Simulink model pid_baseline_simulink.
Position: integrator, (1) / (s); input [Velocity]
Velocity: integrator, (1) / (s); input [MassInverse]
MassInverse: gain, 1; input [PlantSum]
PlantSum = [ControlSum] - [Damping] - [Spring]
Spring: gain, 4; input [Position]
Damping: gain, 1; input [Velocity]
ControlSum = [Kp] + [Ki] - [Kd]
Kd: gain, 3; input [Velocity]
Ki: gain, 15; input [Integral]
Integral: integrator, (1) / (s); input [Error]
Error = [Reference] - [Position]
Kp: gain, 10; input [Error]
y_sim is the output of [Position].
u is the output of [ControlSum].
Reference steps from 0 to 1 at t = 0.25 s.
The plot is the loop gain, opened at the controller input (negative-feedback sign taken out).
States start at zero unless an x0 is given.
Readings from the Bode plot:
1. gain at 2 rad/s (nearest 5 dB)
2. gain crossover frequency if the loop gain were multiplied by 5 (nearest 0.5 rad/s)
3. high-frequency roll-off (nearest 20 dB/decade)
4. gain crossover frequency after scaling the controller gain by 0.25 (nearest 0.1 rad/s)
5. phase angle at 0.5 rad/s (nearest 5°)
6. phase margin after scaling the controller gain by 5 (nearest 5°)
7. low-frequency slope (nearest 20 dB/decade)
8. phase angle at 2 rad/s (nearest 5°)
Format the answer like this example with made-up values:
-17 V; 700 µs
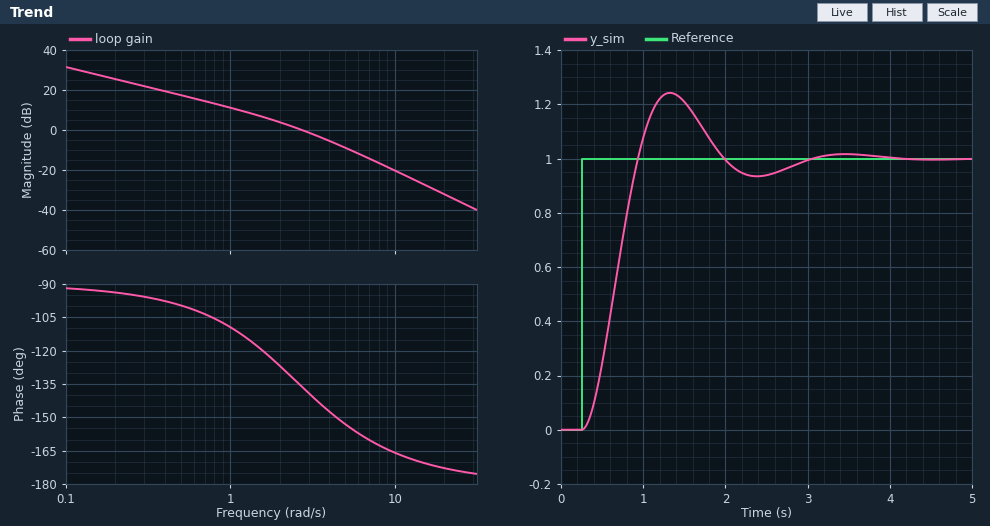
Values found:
5 dB; 7.0 rad/s; -40 dB/decade; 0.9 rad/s; -100°; 20°; -20 dB/decade; -125°
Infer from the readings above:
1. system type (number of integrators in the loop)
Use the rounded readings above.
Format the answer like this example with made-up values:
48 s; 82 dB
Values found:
1
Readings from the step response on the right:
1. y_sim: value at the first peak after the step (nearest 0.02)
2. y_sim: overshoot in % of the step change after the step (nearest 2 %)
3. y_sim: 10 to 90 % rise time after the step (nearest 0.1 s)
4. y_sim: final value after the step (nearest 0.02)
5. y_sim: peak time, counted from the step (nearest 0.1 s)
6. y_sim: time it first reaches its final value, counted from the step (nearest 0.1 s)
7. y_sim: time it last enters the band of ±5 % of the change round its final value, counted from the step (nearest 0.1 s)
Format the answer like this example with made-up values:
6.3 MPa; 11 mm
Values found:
1.24; 24 %; 0.5 s; 1.00; 1.1 s; 0.7 s; 2.4 s
